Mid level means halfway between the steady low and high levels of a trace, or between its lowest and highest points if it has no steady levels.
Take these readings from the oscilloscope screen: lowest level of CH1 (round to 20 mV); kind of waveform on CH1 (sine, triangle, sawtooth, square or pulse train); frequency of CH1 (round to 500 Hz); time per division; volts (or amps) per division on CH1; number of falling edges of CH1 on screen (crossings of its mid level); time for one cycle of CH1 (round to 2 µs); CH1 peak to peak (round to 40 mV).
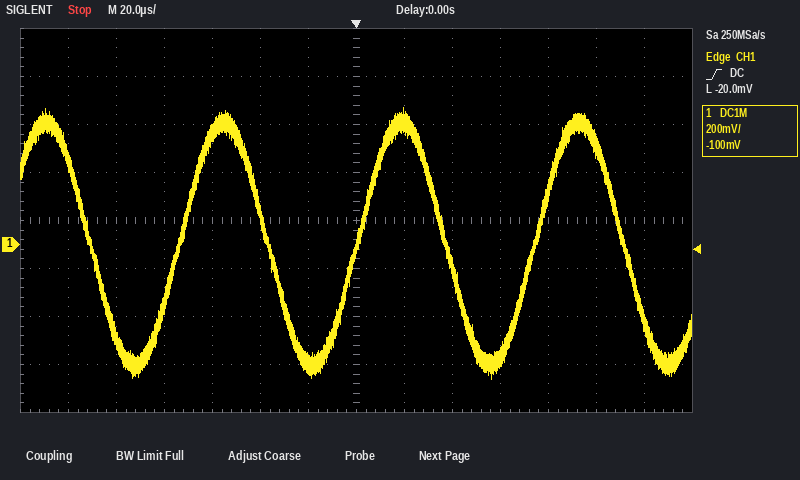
-560 mV
sine
13.5 kHz
20 µs
200 mV
4
74 µs
1.12 V
